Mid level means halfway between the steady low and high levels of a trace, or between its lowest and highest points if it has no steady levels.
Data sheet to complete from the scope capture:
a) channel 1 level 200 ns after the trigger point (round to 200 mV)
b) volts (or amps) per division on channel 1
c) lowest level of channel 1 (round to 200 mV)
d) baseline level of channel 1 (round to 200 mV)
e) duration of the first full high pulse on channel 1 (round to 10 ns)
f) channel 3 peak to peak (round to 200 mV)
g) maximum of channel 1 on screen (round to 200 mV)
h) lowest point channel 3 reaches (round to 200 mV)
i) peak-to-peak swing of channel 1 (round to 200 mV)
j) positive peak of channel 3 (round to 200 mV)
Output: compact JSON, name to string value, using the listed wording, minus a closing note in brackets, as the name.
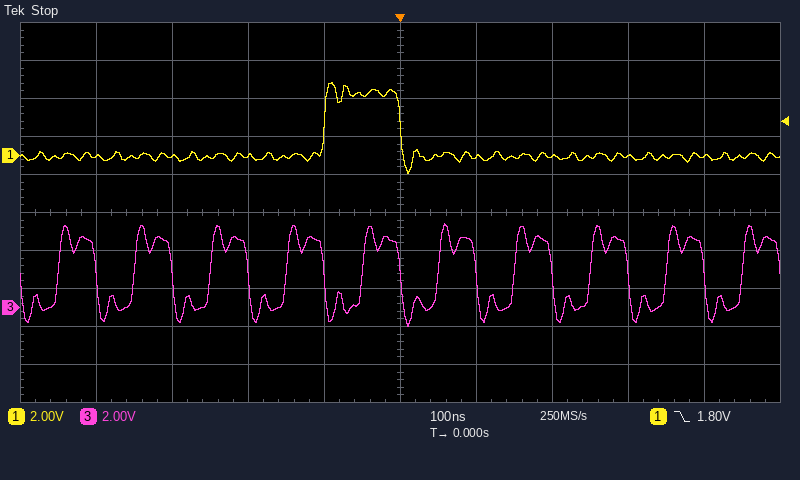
{"channel 1 level 200 ns after the trigger point": "0.0 V", "volts (or amps) per division on channel 1": "2 V", "lowest level of channel 1": "-1.0 V", "baseline level of channel 1": "0.0 V", "duration of the first full high pulse on channel 1": "100 ns", "channel 3 peak to peak": "5.4 V", "maximum of channel 1 on screen": "3.8 V", "lowest point channel 3 reaches": "-1.0 V", "peak-to-peak swing of channel 1": "4.8 V", "positive peak of channel 3": "4.4 V"}
